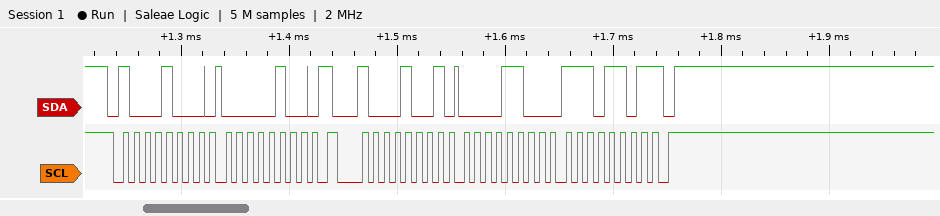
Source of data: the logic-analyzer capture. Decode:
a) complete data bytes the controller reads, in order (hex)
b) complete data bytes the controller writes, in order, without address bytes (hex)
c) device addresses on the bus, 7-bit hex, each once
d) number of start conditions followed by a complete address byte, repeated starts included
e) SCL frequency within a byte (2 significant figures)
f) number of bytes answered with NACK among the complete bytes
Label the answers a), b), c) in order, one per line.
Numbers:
a) 0C ED
b) 04
c) 0x44
d) 2
e) 100 kHz
f) 1
